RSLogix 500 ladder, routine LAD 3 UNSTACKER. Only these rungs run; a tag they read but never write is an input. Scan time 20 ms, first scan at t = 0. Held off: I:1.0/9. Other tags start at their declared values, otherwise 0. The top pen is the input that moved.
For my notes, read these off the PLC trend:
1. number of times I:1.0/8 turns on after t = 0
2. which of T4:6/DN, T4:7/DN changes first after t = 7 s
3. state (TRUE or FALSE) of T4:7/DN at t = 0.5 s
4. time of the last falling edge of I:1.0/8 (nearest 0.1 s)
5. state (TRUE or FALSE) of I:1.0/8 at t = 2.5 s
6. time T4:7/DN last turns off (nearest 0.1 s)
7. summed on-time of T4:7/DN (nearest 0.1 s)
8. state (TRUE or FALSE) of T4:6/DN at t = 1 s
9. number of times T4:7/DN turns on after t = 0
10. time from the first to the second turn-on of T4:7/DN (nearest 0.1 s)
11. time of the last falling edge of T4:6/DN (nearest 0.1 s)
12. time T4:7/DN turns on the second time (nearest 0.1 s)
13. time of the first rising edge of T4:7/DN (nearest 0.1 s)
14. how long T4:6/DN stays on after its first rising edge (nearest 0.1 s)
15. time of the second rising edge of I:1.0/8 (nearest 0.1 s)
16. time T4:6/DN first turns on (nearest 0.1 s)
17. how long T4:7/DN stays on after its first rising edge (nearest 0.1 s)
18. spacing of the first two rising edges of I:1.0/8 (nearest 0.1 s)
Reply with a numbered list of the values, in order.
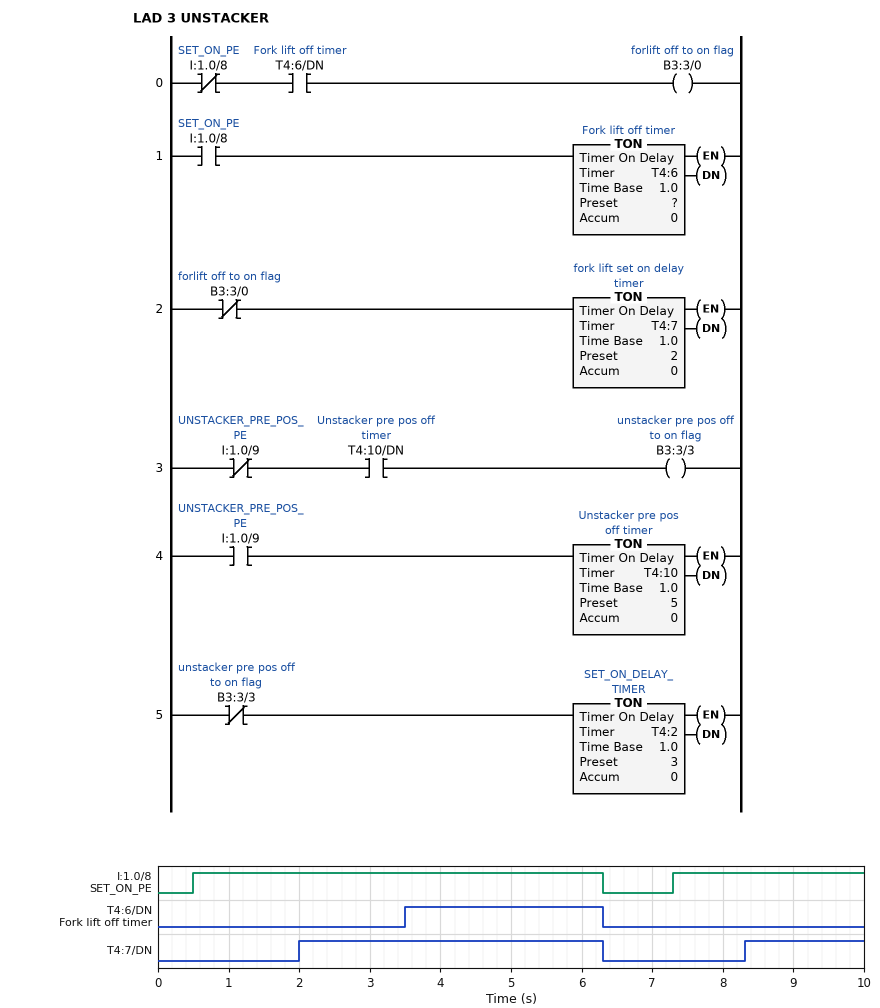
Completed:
1. 2
2. T4:7/DN
3. FALSE
4. 6.3 s
5. TRUE
6. 6.3 s
7. 6.0 s
8. FALSE
9. 2
10. 6.3 s
11. 6.3 s
12. 8.3 s
13. 2.0 s
14. 2.8 s
15. 7.3 s
16. 3.5 s
17. 4.3 s
18. 6.8 s
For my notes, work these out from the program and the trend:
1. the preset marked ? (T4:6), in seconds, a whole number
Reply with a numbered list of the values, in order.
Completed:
1. 3 s
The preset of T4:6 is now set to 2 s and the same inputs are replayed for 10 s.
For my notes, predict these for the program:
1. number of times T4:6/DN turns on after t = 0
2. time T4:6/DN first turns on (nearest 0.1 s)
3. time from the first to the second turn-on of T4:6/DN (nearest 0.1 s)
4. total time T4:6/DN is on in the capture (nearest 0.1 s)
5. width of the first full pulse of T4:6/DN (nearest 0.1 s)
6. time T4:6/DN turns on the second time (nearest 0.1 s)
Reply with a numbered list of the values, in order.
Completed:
1. 2
2. 2.5 s
3. 6.8 s
4. 4.5 s
5. 3.8 s
6. 9.3 s
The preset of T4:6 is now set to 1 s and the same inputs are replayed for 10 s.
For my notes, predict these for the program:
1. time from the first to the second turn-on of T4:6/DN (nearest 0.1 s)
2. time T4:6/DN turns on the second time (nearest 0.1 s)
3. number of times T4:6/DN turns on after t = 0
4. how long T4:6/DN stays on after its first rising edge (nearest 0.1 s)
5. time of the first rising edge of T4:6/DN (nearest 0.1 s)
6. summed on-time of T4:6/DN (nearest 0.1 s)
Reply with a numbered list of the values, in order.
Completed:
1. 6.8 s
2. 8.3 s
3. 2
4. 4.8 s
5. 1.5 s
6. 6.5 s
